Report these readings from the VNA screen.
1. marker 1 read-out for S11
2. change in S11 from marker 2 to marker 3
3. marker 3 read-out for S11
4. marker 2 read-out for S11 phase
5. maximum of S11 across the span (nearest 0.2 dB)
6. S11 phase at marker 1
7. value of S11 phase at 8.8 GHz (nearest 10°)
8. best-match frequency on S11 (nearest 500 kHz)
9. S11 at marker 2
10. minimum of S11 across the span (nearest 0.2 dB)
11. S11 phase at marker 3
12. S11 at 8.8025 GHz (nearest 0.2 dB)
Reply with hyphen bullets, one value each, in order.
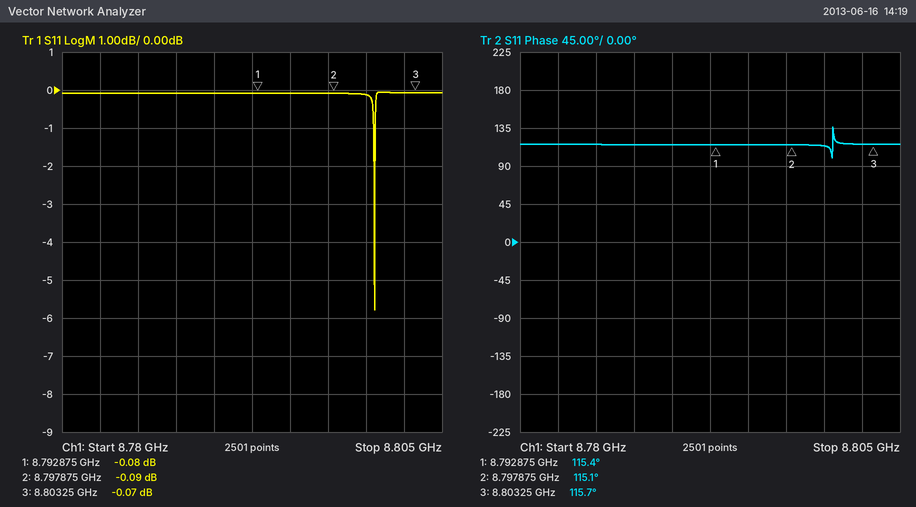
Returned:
- -0.08 dB
- 0.02 dB
- -0.07 dB
- 115.1°
- 0.0 dB
- 115.4°
- 110°
- 8.8005 GHz
- -0.09 dB
- -5.8 dB
- 115.7°
- 0.0 dB
